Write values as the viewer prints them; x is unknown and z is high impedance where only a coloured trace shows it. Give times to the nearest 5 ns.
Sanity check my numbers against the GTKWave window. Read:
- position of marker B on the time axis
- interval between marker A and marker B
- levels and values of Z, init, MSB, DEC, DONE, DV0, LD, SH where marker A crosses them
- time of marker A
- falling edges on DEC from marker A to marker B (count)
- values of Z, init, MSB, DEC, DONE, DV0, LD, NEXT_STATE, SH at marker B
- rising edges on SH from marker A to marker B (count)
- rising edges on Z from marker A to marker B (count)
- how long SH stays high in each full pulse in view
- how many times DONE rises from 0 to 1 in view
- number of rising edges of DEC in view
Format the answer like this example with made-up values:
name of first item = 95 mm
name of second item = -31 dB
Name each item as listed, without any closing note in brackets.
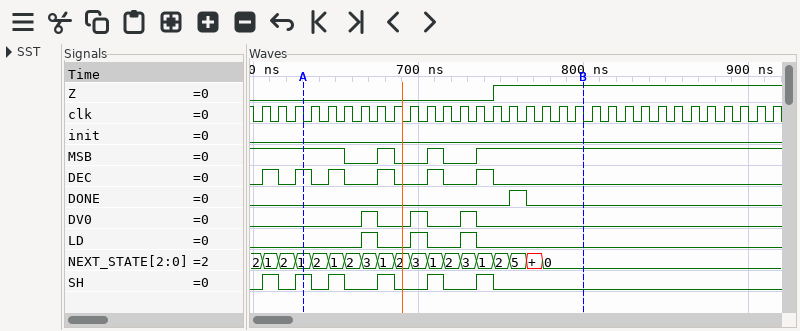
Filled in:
position of marker B on the time axis = 800 ns
interval between marker A and marker B = 170 ns
levels and values of Z, init, MSB, DEC, DONE, DV0, LD, SH where marker A crosses them = Z=0, init=0, MSB=1, DEC=1, DONE=0, DV0=0, LD=0, SH=1
time of marker A = 630 ns
falling edges on DEC from marker A to marker B = 5
values of Z, init, MSB, DEC, DONE, DV0, LD, NEXT_STATE, SH at marker B = Z=1, init=0, MSB=1, DEC=0, DONE=0, DV0=0, LD=0, NEXT_STATE=0, SH=0
rising edges on SH from marker A to marker B = 4
rising edges on Z from marker A to marker B = 1
how long SH stays high in each full pulse in view = 10 ns, 10 ns, 10 ns, 10 ns, 10 ns, 10 ns
how many times DONE rises from 0 to 1 in view = 1
number of rising edges of DEC in view = 6
